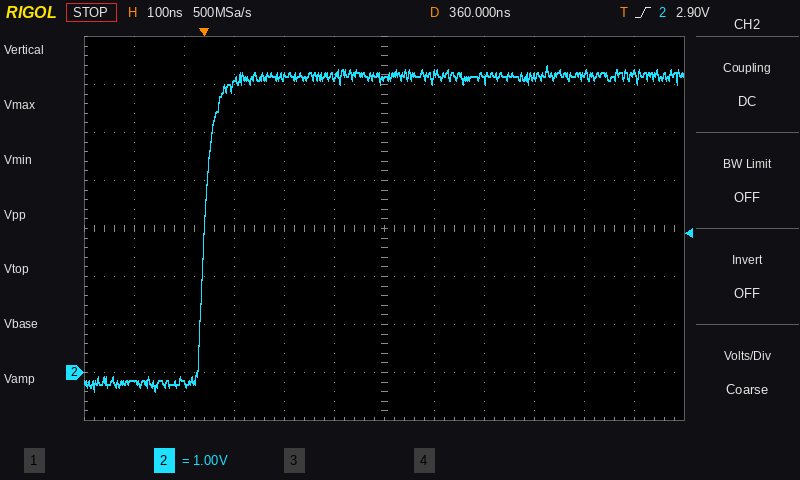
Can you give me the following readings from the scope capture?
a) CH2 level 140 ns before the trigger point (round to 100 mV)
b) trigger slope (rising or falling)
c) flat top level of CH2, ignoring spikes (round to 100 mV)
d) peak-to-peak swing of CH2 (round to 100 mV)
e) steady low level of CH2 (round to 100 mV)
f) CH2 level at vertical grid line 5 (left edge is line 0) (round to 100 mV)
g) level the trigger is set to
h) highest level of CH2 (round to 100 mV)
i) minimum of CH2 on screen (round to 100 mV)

-200 mV
rising
6.2 V
6.8 V
-200 mV
6.2 V
2.90 V
6.4 V
-400 mV
